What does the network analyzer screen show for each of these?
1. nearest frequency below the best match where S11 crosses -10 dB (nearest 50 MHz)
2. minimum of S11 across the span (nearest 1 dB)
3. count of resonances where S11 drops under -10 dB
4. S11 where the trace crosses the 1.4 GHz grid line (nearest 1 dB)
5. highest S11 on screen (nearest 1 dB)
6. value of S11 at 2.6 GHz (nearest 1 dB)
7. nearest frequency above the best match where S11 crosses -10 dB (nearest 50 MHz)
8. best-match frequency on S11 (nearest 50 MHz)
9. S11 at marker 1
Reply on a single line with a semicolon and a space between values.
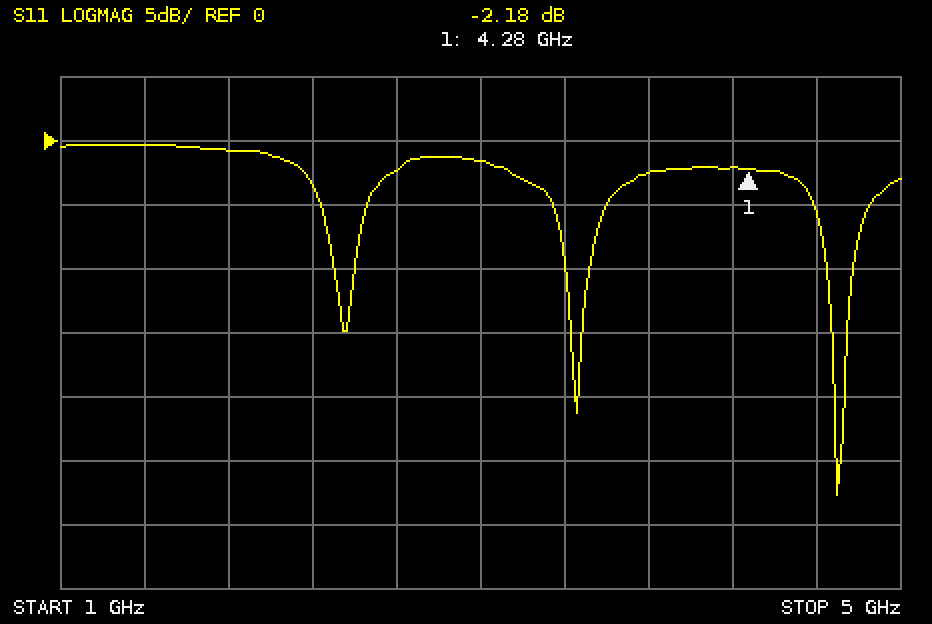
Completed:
4.65 GHz; -28 dB; 3; 0 dB; 0 dB; -2 dB; 4.75 GHz; 4.70 GHz; -2.18 dB
